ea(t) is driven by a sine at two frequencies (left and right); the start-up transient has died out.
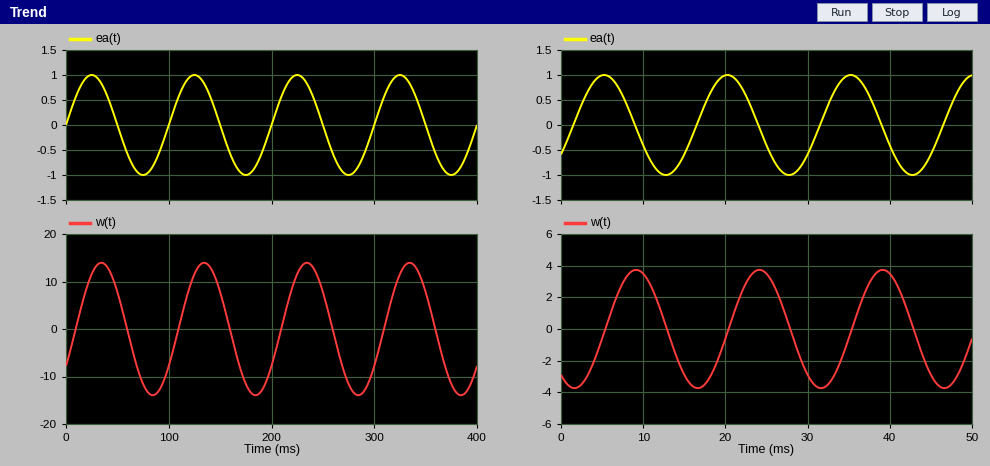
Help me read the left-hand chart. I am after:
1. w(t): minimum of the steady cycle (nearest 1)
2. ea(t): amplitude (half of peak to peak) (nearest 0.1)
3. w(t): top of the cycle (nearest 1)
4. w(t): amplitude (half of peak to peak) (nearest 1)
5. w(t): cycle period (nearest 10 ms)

-14
1.0
14
14
100 ms
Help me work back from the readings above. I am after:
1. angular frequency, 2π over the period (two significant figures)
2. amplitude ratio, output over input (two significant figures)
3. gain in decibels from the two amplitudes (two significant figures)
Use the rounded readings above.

0.063 rad/ms
14
23 dB
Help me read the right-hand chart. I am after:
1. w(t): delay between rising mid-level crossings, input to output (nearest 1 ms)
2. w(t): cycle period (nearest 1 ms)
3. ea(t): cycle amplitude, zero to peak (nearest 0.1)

4 ms
15 ms
1.0
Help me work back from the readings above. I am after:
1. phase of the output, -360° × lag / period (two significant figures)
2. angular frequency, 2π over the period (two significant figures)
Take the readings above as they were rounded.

-96°
0.42 rad/ms
